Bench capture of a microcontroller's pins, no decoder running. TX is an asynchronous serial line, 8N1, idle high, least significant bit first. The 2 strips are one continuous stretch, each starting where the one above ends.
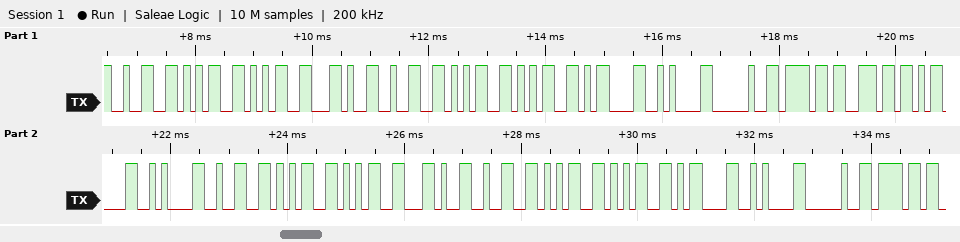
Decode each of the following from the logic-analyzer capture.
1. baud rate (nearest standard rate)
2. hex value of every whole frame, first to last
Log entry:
9600 baud
0x32 0x35 0x35 0x2C 0x32 0x35 0x35 0x0D 0x0A 0x20 0x6F 0x6E 0x0D 0x0A 0x32 0x35 0x35 0x2C 0x32 0x35 0x35 0x0D 0x0A 0x20 0x6F
